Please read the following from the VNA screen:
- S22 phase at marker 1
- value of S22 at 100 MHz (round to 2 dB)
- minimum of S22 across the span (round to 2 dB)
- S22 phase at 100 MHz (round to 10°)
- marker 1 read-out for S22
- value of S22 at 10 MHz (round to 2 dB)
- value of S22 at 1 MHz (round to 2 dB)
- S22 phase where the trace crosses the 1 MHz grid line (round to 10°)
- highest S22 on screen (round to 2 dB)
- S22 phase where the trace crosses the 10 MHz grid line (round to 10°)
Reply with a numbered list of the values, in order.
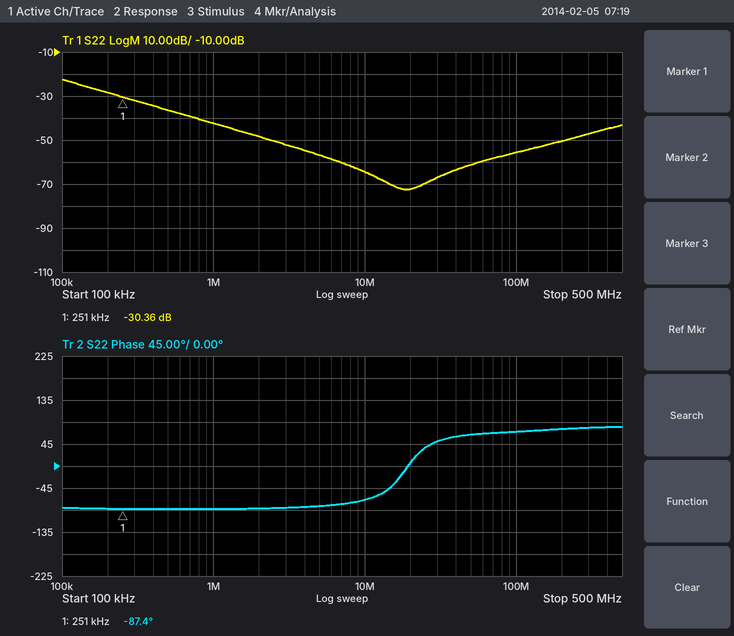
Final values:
1. -87.4°
2. -56 dB
3. -72 dB
4. 70°
5. -30.36 dB
6. -64 dB
7. -42 dB
8. -90°
9. -22 dB
10. -70°
